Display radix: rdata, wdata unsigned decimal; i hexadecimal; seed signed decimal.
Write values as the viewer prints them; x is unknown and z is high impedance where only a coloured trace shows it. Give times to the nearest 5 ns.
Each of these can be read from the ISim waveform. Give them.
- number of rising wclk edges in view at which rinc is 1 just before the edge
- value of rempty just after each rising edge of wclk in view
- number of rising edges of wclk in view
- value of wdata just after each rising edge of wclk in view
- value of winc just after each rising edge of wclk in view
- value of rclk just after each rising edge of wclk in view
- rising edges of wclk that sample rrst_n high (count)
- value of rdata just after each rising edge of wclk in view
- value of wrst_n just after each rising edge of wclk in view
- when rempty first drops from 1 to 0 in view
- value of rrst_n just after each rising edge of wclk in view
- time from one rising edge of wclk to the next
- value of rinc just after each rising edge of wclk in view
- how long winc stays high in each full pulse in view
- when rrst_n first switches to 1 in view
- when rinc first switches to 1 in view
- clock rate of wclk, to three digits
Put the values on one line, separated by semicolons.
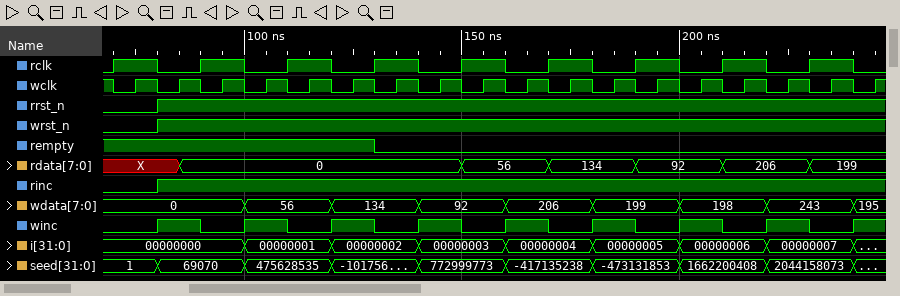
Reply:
17; 1 1 1 1 1 1 0 0 0 0 0 0 0 0 0 0 0 0; 18; 0, 0, 0, 56, 56, 134, 134, 92, 92, 206, 206, 199, 199, 198, 198, 243, 243, 195; 0 1 0 1 0 1 0 1 0 1 0 1 0 1 0 1 0 1; 1 0 1 0 1 0 1 0 1 0 1 0 1 0 1 0 1 0; 17; X, 0, 0, 0, 0, 0, 0, 0, 56, 56, 134, 134, 92, 92, 206, 206, 199, 199; 0 1 1 1 1 1 1 1 1 1 1 1 1 1 1 1 1 1; 130 ns; 0 1 1 1 1 1 1 1 1 1 1 1 1 1 1 1 1 1; 10 ns; 0 1 1 1 1 1 1 1 1 1 1 1 1 1 1 1 1 1; 10 ns, 10 ns, 10 ns, 10 ns, 10 ns, 10 ns, 10 ns, 10 ns; 80 ns; 80 ns; 100 MHz
